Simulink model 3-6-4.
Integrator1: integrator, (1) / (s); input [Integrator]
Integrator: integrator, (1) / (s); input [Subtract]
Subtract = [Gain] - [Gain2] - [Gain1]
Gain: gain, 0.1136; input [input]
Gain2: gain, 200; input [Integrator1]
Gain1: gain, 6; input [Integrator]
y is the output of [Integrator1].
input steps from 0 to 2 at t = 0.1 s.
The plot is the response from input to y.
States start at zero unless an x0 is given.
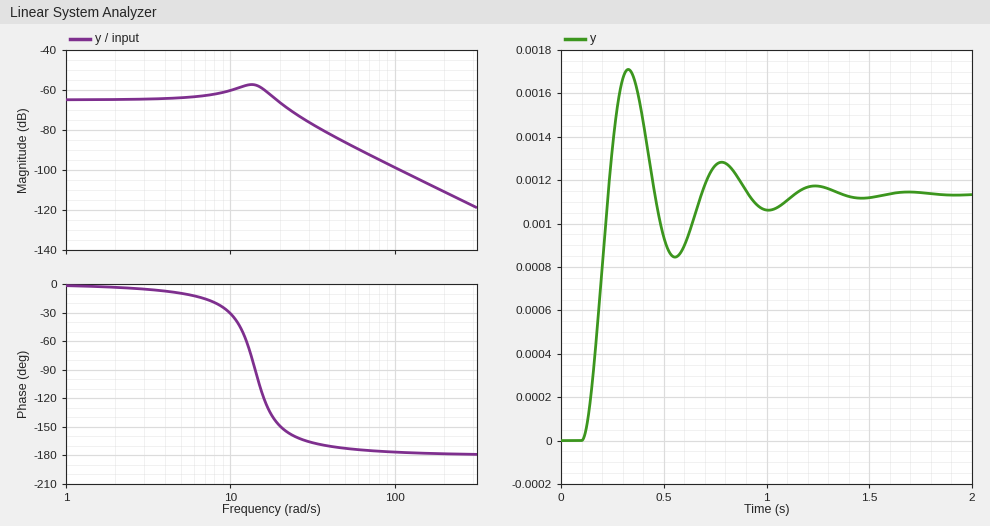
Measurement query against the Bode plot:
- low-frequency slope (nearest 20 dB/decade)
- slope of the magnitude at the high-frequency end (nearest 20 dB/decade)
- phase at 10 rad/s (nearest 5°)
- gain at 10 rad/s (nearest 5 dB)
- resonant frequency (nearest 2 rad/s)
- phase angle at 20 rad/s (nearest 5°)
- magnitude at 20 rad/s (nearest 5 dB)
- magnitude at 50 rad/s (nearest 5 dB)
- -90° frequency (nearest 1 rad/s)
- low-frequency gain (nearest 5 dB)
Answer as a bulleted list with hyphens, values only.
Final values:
- 0 dB/decade
- -40 dB/decade
- -30°
- -60 dB
- 14 rad/s
- -150°
- -65 dB
- -85 dB
- 14 rad/s
- -65 dB
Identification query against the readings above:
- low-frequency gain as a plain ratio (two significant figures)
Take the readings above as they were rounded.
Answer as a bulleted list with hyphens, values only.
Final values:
- 0.00056
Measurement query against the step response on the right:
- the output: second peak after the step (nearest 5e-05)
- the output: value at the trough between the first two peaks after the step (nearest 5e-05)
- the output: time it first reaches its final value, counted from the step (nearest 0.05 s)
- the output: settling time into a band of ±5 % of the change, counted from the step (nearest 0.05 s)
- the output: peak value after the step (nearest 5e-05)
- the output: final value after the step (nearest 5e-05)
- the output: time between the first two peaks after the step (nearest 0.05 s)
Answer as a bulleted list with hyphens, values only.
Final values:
- 0.00130
- 0.00085
- 0.15 s
- 0.95 s
- 0.00170
- 0.00115
- 0.45 s
